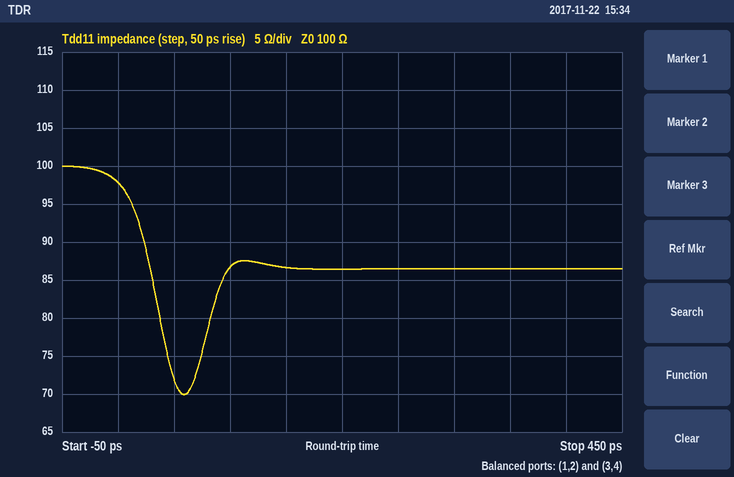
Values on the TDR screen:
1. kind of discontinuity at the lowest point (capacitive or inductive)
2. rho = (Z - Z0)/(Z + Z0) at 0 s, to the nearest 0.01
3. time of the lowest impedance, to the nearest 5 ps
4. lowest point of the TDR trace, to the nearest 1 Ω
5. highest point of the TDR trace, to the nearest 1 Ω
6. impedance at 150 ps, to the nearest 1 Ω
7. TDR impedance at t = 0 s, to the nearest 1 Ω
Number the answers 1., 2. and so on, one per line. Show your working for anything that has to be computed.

1. capacitive
2. (98 − 100)/(98 + 100) ≈ -0.01
3. 60 ps
4. 70 Ω
5. 100 Ω
6. 87 Ω
7. 98 Ω
